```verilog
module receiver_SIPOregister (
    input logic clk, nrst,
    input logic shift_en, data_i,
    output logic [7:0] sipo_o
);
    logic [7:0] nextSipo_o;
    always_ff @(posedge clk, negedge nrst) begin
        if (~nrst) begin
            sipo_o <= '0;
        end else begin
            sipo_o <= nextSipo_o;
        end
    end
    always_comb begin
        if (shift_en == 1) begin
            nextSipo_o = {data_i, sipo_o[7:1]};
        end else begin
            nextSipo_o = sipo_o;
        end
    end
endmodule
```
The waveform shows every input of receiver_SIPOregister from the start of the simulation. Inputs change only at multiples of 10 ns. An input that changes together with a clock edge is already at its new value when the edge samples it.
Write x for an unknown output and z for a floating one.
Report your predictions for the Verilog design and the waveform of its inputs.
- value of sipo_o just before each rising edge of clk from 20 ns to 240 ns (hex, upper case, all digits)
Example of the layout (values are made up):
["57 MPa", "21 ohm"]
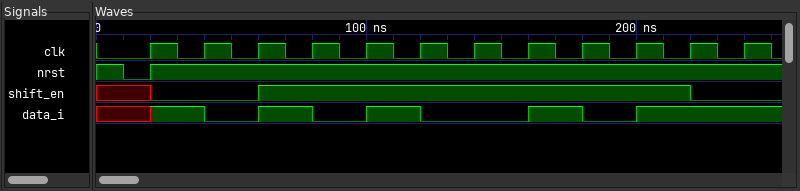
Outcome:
["00, 00, 00, 80, 40, A0, 50, 28, 94, 4A, A5, A5"]
